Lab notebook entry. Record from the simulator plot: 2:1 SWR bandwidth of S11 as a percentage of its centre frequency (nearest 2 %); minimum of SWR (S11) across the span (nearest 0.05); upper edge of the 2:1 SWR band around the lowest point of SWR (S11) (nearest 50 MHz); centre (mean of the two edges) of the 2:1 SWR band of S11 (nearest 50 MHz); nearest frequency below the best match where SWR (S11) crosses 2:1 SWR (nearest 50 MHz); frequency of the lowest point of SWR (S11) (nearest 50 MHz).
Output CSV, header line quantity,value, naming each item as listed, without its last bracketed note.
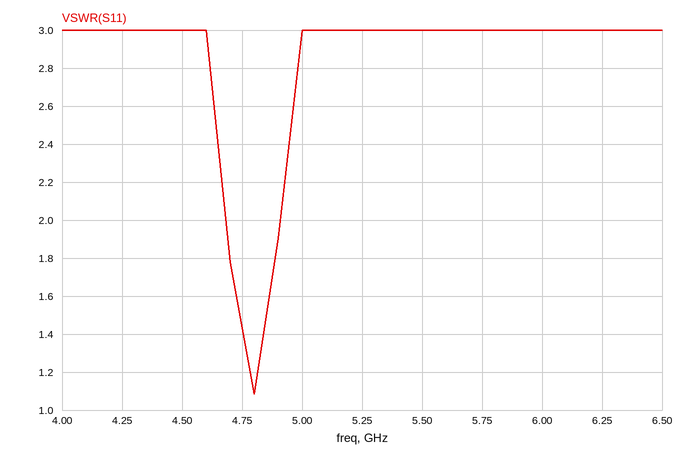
quantity,value
2:1 SWR bandwidth of S11 as a percentage of its centre frequency,4 %
minimum of SWR (S11) across the span,1.10
upper edge of the 2:1 SWR band around the lowest point of SWR (S11),4.90 GHz
centre (mean of the two edges) of the 2:1 SWR band of S11,4.80 GHz
nearest frequency below the best match where SWR (S11) crosses 2:1 SWR,4.70 GHz
frequency of the lowest point of SWR (S11),4.80 GHz
